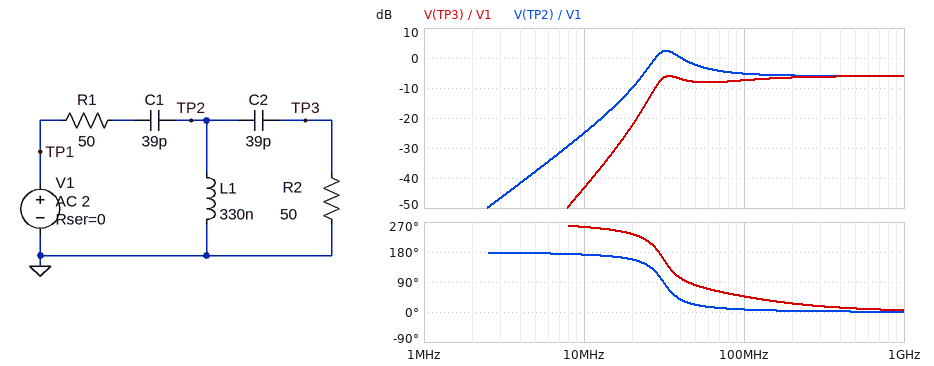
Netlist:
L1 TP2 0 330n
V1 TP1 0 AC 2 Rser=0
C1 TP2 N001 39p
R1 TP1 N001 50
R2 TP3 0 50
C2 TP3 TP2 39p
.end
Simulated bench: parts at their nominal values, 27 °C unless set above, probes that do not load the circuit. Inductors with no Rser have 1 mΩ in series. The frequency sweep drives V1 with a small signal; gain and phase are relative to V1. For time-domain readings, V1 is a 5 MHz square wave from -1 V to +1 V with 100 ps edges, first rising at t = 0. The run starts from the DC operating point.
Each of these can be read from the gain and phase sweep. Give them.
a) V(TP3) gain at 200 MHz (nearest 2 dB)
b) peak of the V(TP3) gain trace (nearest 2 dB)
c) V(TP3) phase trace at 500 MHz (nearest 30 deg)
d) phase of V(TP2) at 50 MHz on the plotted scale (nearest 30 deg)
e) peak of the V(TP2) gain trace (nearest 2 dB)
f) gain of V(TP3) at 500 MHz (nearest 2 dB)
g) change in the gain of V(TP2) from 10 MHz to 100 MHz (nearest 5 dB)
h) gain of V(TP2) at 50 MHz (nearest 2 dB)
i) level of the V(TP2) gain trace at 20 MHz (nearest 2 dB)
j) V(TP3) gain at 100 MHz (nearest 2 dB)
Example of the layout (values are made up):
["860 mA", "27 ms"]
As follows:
["-6 dB", "-6 dB", "0 deg", "30 deg", "2 dB", "-6 dB", "20 dB", "-2 dB", "-10 dB", "-8 dB"]
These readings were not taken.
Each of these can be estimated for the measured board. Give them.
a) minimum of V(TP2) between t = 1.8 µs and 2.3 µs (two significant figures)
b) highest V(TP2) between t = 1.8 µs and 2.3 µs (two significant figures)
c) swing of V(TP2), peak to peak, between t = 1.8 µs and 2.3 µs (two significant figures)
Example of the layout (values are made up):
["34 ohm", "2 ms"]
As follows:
["-980 mV", "980 mV", "2.0 V"]
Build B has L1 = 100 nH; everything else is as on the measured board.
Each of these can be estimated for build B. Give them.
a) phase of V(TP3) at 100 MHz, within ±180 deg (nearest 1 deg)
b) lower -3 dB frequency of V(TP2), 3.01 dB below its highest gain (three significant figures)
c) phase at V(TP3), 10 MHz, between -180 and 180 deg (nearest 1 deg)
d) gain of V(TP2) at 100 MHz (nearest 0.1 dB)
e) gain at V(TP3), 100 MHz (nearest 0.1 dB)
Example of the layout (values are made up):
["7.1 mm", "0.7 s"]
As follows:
["70 deg", "48.0 MHz", "-104 deg", "-3.9 dB", "-6.1 dB"]
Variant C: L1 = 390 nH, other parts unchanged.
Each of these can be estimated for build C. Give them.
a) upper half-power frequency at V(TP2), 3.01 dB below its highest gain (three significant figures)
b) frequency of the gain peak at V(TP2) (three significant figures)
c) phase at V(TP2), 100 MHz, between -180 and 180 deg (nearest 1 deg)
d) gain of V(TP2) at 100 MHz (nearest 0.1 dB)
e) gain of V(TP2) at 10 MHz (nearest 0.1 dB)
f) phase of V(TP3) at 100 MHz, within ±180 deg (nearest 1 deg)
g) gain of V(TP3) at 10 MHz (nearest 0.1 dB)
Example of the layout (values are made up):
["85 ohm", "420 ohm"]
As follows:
["37.6 MHz", "29.8 MHz", "6 deg", "-5.3 dB", "-23.4 dB", "46 deg", "-41.7 dB"]
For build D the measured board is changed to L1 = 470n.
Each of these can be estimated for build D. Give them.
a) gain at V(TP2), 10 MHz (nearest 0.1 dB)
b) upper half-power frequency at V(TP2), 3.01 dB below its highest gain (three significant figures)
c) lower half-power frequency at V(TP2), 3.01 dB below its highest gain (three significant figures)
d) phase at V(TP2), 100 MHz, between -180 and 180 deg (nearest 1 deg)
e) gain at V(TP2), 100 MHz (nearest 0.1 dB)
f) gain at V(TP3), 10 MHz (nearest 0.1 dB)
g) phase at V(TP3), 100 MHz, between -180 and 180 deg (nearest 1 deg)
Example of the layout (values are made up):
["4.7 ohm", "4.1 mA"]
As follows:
["-21.5 dB", "33.1 MHz", "23.4 MHz", "5 deg", "-5.4 dB", "-39.8 dB", "44 deg"]
